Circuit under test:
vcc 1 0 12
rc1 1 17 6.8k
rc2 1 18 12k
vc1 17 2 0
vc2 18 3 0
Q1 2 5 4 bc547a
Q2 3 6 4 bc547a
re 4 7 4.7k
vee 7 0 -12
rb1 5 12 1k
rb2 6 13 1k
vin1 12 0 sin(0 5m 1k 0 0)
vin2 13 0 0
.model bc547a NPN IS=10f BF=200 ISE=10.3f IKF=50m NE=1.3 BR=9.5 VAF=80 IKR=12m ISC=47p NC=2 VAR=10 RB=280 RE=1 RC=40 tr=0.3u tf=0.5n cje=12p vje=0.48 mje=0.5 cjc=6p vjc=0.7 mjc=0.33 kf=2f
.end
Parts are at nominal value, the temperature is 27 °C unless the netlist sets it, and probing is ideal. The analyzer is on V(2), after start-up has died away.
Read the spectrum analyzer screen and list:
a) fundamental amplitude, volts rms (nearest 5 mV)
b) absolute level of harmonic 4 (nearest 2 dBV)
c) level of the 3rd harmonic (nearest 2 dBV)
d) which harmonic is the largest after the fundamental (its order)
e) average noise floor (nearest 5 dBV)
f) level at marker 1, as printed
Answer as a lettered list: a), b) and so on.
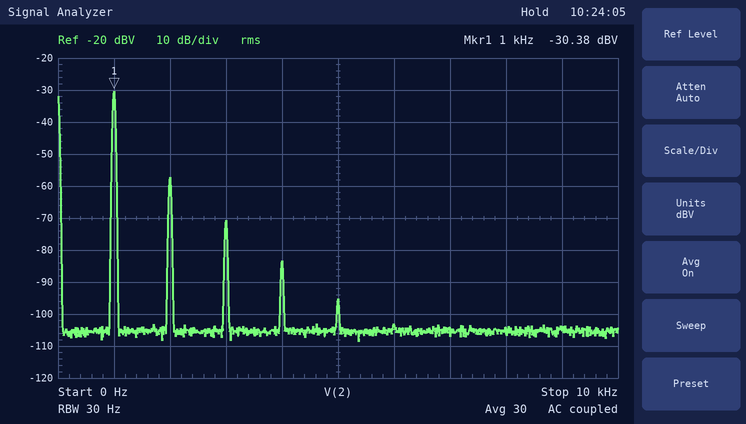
a) 30 mV
b) -84 dBV
c) -70 dBV
d) 2
e) -105 dBV
f) -30.38 dBV
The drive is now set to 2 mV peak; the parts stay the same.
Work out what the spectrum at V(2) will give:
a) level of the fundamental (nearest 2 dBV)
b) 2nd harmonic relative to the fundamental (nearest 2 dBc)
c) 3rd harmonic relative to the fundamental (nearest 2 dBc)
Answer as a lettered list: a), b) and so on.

a) -38 dBV
b) -36 dBc
c) -58 dBc
